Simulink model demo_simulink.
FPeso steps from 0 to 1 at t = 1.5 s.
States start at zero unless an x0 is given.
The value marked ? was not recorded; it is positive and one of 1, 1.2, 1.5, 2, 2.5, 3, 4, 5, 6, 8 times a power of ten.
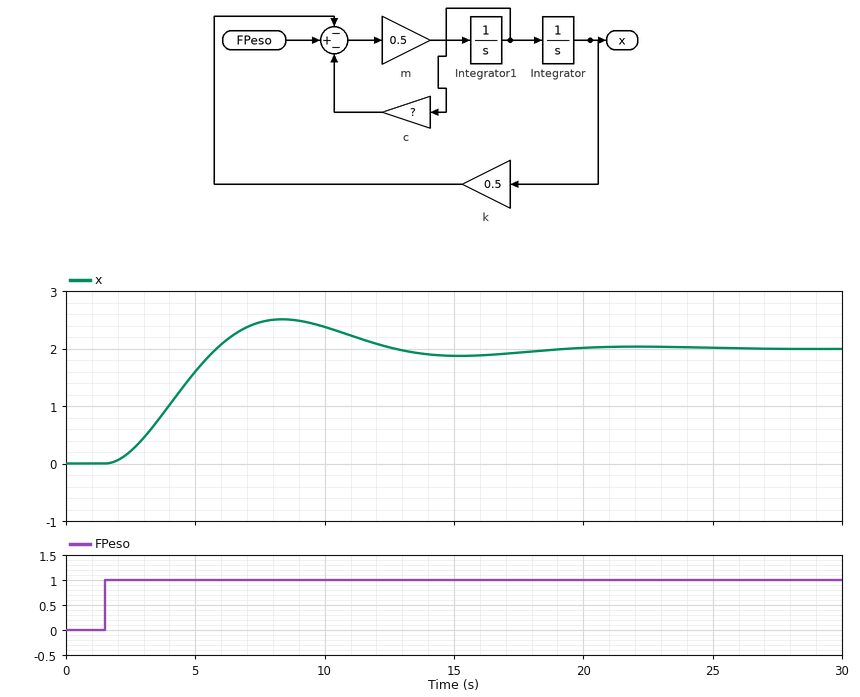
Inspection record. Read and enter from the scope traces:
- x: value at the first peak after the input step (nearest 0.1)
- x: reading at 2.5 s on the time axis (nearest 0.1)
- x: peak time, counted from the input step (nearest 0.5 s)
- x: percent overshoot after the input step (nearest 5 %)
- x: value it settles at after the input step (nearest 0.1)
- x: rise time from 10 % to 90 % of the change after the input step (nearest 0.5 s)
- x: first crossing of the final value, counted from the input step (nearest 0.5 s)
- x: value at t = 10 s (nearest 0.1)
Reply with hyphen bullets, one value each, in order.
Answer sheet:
- 2.5
- 0.2
- 7.0 s
- 25 %
- 2.0
- 3.0 s
- 4.5 s
- 2.4
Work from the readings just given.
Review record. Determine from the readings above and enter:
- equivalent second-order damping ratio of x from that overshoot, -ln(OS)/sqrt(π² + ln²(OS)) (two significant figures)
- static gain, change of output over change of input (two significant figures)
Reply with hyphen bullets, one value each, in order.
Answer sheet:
- 0.40
- 2.0
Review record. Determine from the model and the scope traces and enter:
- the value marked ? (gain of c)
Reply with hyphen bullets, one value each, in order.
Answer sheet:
- 0.8
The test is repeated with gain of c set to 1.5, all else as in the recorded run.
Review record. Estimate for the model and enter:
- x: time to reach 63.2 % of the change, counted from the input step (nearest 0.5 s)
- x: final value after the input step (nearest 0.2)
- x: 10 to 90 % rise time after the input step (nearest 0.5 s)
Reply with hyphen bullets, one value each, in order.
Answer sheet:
- 3.5 s
- 2.0
- 4.5 s
